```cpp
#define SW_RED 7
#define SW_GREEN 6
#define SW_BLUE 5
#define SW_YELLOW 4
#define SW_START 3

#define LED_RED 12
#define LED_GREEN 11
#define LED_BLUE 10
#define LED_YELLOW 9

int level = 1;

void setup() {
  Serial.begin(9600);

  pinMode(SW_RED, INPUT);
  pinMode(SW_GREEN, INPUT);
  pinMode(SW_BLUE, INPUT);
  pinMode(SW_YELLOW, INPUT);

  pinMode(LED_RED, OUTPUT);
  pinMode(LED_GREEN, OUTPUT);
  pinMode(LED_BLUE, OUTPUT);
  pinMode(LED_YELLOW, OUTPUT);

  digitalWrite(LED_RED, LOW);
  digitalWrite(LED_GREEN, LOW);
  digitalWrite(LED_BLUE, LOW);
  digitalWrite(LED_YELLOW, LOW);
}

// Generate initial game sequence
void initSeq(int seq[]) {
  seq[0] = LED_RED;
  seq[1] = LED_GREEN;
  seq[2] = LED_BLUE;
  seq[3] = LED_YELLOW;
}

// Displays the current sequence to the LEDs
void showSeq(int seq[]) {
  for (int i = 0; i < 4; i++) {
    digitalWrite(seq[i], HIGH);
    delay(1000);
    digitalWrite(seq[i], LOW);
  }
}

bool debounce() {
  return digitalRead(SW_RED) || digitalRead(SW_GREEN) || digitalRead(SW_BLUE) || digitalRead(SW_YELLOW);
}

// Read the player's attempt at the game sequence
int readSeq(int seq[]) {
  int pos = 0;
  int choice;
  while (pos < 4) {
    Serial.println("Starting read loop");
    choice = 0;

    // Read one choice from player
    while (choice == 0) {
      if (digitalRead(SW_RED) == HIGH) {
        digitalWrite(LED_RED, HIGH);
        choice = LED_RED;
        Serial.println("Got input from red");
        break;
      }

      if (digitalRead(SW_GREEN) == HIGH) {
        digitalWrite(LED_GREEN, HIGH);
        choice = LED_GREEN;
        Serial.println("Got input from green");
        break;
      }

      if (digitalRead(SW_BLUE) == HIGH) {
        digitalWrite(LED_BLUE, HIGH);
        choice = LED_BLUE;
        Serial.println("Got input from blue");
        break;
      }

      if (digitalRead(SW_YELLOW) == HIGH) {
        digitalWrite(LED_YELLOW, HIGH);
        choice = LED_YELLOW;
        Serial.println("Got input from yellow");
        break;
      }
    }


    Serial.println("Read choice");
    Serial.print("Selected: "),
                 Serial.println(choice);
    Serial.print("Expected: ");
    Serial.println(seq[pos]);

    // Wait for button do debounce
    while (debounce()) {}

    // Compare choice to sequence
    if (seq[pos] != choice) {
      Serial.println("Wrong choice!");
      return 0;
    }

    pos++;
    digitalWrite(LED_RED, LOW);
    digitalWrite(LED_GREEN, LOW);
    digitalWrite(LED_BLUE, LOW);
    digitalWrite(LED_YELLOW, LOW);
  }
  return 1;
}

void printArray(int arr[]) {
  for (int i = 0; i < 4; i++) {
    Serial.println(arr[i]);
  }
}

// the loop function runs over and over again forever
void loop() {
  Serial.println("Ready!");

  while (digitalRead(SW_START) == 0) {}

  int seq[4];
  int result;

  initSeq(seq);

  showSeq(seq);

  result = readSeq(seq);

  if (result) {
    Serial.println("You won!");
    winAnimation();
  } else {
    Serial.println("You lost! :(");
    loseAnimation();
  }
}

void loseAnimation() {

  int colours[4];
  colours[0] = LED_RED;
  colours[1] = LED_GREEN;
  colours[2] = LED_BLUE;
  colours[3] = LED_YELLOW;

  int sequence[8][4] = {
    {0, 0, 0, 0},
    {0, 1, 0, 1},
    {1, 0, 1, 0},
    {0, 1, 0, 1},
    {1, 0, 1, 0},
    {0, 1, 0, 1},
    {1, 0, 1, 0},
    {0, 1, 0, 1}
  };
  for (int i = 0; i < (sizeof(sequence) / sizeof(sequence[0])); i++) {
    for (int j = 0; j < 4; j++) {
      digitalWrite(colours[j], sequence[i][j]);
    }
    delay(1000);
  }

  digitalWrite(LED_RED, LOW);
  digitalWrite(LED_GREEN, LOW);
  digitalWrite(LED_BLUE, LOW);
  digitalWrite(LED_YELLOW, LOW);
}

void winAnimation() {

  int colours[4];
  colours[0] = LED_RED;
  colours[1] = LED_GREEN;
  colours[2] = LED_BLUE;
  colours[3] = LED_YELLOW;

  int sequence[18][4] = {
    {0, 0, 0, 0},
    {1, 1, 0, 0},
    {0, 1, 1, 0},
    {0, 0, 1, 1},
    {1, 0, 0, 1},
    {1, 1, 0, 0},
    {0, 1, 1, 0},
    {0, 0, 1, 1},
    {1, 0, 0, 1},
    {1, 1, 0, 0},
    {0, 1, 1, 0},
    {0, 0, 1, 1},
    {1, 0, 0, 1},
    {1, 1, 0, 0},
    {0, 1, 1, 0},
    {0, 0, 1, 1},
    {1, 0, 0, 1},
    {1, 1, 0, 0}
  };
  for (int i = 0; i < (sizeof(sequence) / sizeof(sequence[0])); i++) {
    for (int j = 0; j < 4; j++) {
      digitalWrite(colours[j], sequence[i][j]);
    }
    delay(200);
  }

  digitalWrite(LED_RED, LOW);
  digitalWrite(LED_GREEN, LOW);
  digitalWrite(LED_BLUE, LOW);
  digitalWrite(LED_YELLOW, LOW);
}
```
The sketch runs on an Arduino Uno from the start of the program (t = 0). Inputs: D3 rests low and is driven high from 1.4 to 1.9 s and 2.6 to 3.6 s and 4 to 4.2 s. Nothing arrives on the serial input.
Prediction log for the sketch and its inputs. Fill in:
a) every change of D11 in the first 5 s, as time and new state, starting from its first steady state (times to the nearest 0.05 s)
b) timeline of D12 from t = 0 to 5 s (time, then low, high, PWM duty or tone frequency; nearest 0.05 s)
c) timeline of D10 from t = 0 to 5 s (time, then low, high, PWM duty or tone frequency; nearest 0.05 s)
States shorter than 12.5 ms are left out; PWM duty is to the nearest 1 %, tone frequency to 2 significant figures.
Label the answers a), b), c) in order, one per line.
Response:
a) 0 s low; 2.4 s high; 3.4 s low
b) 0 s low; 1.4 s high; 2.4 s low
c) 0 s low; 3.4 s high; 4.4 s low
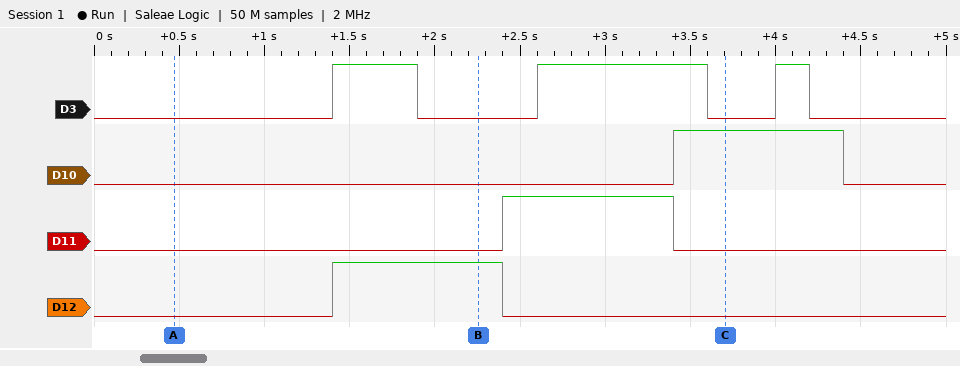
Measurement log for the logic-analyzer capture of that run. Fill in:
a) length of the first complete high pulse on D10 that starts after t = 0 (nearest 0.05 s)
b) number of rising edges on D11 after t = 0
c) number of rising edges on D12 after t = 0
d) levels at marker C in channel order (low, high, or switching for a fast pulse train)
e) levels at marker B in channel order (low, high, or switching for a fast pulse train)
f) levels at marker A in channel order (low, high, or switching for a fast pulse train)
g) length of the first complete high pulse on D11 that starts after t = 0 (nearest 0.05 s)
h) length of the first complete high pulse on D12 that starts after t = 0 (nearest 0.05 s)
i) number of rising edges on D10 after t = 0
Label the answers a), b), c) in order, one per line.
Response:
a) 1.00 s
b) 1
c) 1
d) D3 low, D10 high, D11 low, D12 low
e) D3 low, D10 low, D11 low, D12 high
f) D3 low, D10 low, D11 low, D12 low
g) 1.00 s
h) 1.00 s
i) 1
